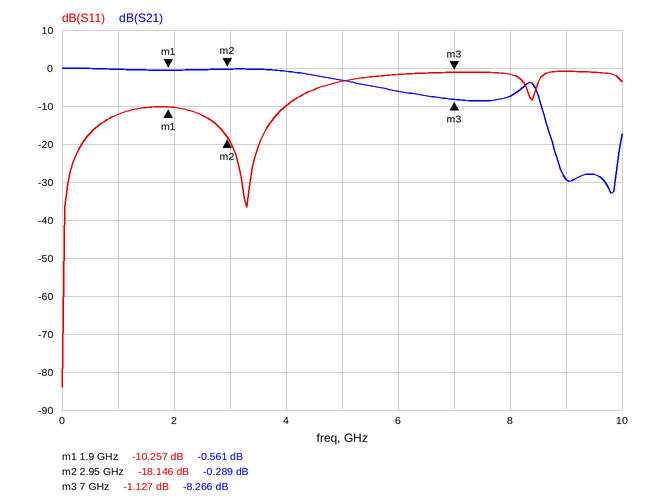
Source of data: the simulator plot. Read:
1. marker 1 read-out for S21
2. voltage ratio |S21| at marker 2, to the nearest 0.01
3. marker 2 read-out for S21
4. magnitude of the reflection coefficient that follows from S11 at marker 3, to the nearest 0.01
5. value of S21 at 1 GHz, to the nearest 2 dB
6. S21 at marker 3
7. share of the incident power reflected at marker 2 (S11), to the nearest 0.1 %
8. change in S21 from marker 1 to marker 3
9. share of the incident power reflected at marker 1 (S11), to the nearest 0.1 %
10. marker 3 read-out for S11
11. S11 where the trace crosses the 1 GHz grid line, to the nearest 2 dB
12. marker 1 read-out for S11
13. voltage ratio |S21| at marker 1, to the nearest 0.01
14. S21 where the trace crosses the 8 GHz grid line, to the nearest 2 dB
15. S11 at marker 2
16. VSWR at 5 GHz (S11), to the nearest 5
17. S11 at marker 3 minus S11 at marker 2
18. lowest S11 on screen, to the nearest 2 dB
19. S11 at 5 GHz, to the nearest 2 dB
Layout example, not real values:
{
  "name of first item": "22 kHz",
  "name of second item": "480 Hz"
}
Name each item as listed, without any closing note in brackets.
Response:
{
  "marker 1 read-out for S21": "-0.561 dB",
  "voltage ratio |S21| at marker 2, to the nearest 0.01": "0.97",
  "marker 2 read-out for S21": "-0.289 dB",
  "magnitude of the reflection coefficient that follows from S11 at marker 3, to the nearest 0.01": "0.88",
  "value of S21 at 1 GHz, to the nearest 2 dB": "0 dB",
  "S21 at marker 3": "-8.266 dB",
  "share of the incident power reflected at marker 2 (S11), to the nearest 0.1 %": "1.5 %",
  "change in S21 from marker 1 to marker 3": "-7.705 dB",
  "share of the incident power reflected at marker 1 (S11), to the nearest 0.1 %": "9.4 %",
  "marker 3 read-out for S11": "-1.127 dB",
  "S11 where the trace crosses the 1 GHz grid line, to the nearest 2 dB": "-12 dB",
  "marker 1 read-out for S11": "-10.257 dB",
  "voltage ratio |S21| at marker 1, to the nearest 0.01": "0.94",
  "S21 where the trace crosses the 8 GHz grid line, to the nearest 2 dB": "-8 dB",
  "S11 at marker 2": "-18.146 dB",
  "VSWR at 5 GHz (S11), to the nearest 5": "5",
  "S11 at marker 3 minus S11 at marker 2": "17.019 dB",
  "lowest S11 on screen, to the nearest 2 dB": "-84 dB",
  "S11 at 5 GHz, to the nearest 2 dB": "-4 dB"
}
